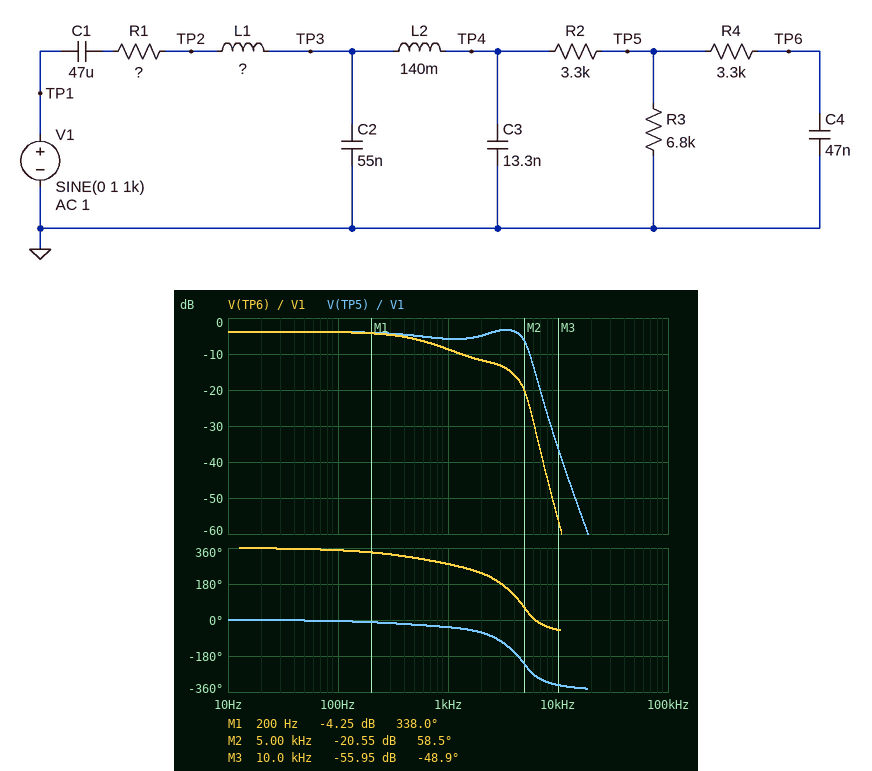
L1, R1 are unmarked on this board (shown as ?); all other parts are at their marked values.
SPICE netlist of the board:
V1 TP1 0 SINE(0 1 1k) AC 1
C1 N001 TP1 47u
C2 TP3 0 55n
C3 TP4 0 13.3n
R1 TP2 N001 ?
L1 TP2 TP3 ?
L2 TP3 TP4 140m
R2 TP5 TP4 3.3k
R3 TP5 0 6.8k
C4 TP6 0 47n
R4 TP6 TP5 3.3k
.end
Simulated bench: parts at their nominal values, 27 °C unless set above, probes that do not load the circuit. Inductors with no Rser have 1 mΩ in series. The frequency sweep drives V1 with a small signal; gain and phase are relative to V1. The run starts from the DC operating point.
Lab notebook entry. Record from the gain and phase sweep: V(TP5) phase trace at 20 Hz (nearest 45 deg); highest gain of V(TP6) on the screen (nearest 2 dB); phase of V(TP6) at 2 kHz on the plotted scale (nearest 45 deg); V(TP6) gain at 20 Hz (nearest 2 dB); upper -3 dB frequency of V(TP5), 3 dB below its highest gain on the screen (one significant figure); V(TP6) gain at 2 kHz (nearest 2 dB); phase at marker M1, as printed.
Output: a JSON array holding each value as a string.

["0 deg", "-4 dB", "225 deg", "-4 dB", "5 kHz", "-12 dB", "338.0 deg"]
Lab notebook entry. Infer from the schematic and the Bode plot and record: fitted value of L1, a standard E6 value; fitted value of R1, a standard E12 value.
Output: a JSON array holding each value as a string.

["22 mH", "470 Ω"]
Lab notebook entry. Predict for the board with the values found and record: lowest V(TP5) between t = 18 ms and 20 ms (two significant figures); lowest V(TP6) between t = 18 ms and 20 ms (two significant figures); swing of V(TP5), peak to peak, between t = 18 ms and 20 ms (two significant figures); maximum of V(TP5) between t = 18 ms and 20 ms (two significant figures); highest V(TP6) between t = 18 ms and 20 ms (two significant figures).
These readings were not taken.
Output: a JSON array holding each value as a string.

["-510 mV", "-370 mV", "1.0 V", "510 mV", "370 mV"]
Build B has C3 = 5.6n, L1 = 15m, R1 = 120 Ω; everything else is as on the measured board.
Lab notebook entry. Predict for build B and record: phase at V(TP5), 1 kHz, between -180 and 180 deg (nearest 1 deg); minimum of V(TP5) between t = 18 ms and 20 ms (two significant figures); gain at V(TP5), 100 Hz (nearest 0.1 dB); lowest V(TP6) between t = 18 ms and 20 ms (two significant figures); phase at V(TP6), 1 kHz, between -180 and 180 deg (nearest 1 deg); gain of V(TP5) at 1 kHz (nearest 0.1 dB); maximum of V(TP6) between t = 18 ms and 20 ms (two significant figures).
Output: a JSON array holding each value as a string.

["-26 deg", "-530 mV", "-3.6 dB", "-380 mV", "-71 deg", "-5.6 dB", "380 mV"]
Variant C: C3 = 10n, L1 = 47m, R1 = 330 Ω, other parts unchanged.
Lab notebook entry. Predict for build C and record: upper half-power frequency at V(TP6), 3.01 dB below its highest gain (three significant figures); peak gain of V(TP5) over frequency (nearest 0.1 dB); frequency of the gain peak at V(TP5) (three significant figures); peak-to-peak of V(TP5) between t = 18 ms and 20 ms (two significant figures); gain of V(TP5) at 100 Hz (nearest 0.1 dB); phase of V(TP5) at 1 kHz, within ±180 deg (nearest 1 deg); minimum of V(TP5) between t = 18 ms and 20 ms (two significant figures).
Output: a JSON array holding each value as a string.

["724 Hz", "-1.3 dB", "2.82 kHz", "1.1 V", "-3.8 dB", "-35 deg", "-560 mV"]
